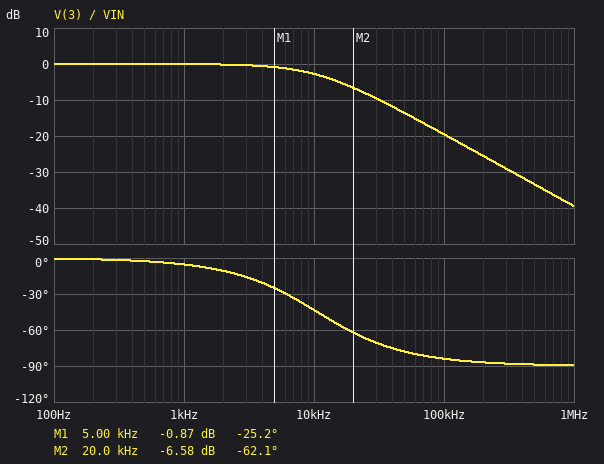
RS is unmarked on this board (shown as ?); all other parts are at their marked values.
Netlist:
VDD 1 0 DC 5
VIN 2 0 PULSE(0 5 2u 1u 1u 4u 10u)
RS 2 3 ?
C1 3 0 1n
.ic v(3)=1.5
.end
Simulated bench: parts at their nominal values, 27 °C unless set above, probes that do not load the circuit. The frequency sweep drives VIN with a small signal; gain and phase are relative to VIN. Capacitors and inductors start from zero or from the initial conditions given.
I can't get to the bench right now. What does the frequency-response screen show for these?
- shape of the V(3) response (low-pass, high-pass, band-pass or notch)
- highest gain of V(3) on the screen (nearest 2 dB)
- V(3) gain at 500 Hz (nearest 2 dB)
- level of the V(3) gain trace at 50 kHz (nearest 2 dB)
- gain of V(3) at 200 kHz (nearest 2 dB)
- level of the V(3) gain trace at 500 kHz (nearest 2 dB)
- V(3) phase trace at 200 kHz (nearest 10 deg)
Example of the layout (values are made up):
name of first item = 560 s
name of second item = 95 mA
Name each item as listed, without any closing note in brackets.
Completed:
shape of the V(3) response = low-pass
highest gain of V(3) on the screen = 0 dB
V(3) gain at 500 Hz = 0 dB
level of the V(3) gain trace at 50 kHz = -14 dB
gain of V(3) at 200 kHz = -26 dB
level of the V(3) gain trace at 500 kHz = -34 dB
V(3) phase trace at 200 kHz = -90 deg
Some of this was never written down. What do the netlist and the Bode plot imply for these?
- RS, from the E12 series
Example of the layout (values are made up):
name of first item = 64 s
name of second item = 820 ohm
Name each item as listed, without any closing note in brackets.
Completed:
RS, from the E12 series = 15 kΩ
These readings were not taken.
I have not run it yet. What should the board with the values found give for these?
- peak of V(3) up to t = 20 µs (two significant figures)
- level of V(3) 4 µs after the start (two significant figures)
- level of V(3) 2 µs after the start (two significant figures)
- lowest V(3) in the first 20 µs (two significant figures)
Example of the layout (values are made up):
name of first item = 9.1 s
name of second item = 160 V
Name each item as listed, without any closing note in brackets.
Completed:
peak of V(3) up to t = 20 µs = 2.6 V
level of V(3) 4 µs after the start = 1.6 V
level of V(3) 2 µs after the start = 1.3 V
lowest V(3) in the first 20 µs = 1.3 V
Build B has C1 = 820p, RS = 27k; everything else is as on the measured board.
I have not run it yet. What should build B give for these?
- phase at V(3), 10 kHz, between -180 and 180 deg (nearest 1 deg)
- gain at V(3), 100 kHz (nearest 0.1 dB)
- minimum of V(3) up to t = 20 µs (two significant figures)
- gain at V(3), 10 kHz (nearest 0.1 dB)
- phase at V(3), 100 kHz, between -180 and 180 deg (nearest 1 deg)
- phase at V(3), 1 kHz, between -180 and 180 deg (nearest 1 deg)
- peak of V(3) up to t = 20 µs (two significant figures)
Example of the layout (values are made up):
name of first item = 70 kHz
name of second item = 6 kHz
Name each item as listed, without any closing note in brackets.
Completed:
phase at V(3), 10 kHz, between -180 and 180 deg = -54 deg
gain at V(3), 100 kHz = -22.9 dB
minimum of V(3) up to t = 20 µs = 1.4 V
gain at V(3), 10 kHz = -4.7 dB
phase at V(3), 100 kHz, between -180 and 180 deg = -86 deg
phase at V(3), 1 kHz, between -180 and 180 deg = -8 deg
peak of V(3) up to t = 20 µs = 2.3 V
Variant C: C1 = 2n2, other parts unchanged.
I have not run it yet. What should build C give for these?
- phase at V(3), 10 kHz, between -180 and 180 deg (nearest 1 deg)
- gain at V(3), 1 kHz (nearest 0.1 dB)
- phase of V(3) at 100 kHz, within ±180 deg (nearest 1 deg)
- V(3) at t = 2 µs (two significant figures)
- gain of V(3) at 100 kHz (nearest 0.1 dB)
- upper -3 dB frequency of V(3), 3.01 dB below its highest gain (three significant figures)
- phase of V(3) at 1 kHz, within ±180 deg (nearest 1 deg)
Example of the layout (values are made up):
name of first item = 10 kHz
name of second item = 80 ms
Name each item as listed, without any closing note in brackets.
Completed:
phase at V(3), 10 kHz, between -180 and 180 deg = -64 deg
gain at V(3), 1 kHz = -0.2 dB
phase of V(3) at 100 kHz, within ±180 deg = -87 deg
V(3) at t = 2 µs = 1.4 V
gain of V(3) at 100 kHz = -26.3 dB
upper -3 dB frequency of V(3), 3.01 dB below its highest gain = 4.82 kHz
phase of V(3) at 1 kHz, within ±180 deg = -12 deg
